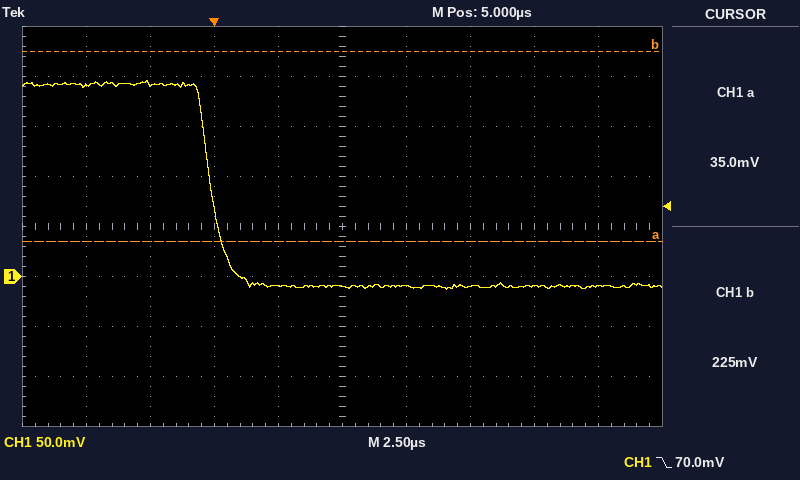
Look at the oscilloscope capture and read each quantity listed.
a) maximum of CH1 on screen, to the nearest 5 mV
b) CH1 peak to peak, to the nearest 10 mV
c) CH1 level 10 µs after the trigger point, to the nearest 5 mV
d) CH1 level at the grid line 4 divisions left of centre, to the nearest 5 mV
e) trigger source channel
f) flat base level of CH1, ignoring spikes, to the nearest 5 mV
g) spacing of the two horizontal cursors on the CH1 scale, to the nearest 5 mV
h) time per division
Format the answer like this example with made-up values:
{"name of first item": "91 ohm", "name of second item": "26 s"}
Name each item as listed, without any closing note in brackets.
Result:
{"maximum of CH1 on screen, to the nearest 5 mV": "195 mV", "CH1 peak to peak, to the nearest 10 mV": "210 mV", "CH1 level 10 µs after the trigger point, to the nearest 5 mV": "-10 mV", "CH1 level at the grid line 4 divisions left of centre, to the nearest 5 mV": "190 mV", "trigger source channel": "CH1", "flat base level of CH1, ignoring spikes, to the nearest 5 mV": "-10 mV", "spacing of the two horizontal cursors on the CH1 scale, to the nearest 5 mV": "190 mV", "time per division": "2.5 µs"}
